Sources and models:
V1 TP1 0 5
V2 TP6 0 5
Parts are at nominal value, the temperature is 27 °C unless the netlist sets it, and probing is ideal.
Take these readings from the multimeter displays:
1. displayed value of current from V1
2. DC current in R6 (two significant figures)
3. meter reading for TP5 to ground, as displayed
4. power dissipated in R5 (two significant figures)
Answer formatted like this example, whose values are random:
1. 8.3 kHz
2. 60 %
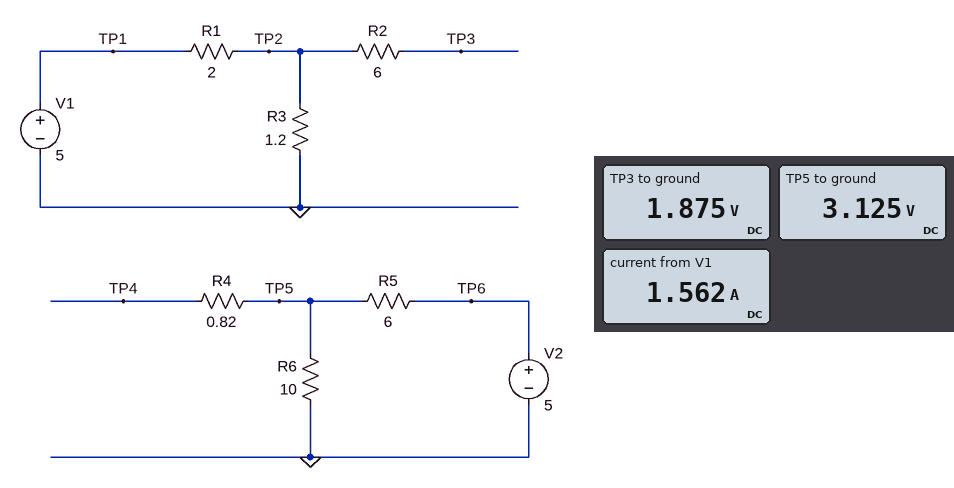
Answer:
1. 1.562 A
2. 310 mA
3. 3.125 V
4. 590 mW
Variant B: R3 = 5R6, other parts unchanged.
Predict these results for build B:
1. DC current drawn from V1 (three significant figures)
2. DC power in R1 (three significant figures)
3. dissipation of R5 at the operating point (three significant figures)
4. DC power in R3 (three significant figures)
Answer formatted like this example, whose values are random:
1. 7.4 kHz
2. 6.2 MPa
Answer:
1. 658 mA
2. 866 mW
3. 586 mW
4. 2.42 W
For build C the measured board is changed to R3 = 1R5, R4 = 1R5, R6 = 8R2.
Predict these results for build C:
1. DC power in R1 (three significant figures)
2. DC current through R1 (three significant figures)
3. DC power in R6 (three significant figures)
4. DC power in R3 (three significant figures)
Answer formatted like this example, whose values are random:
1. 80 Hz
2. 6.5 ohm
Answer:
1. 4.08 W
2. 1.43 A
3. 1.02 W
4. 3.06 W
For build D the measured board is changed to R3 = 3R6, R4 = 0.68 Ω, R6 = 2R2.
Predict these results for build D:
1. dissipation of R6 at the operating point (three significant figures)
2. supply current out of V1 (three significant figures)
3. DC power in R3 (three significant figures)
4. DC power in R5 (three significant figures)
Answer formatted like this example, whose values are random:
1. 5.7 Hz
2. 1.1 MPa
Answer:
1. 818 mW
2. 893 mA
3. 2.87 W
4. 2.23 W
